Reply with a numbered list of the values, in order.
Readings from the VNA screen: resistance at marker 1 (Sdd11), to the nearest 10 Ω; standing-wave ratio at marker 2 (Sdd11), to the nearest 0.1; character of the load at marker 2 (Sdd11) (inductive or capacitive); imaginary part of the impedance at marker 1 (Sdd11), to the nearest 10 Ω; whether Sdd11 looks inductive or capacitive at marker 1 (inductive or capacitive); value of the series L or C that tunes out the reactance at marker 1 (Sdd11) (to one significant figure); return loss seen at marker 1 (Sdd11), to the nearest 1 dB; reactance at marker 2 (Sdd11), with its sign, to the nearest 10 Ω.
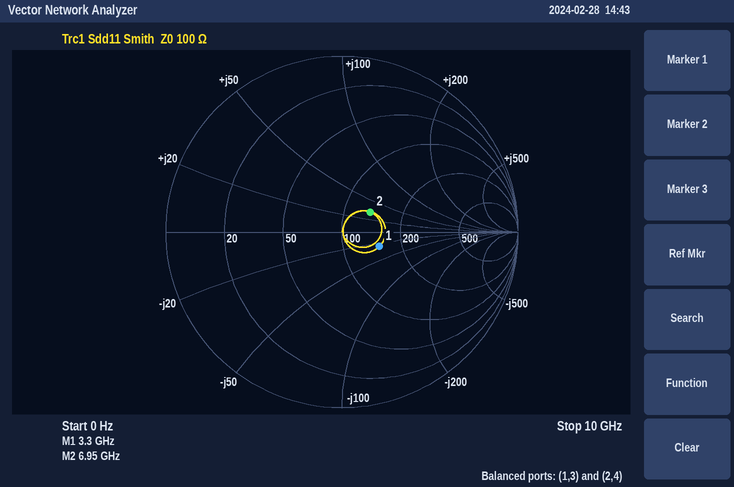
1. 150 Ω
2. 1.5
3. inductive
4. -30 Ω
5. capacitive
6. 1 nH
7. 13 dB
8. +30 Ω
